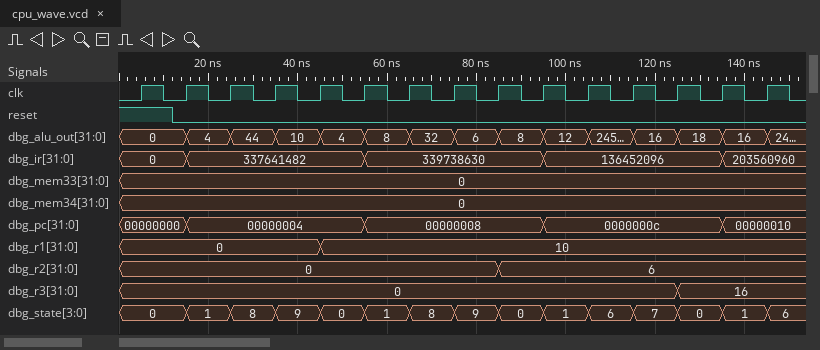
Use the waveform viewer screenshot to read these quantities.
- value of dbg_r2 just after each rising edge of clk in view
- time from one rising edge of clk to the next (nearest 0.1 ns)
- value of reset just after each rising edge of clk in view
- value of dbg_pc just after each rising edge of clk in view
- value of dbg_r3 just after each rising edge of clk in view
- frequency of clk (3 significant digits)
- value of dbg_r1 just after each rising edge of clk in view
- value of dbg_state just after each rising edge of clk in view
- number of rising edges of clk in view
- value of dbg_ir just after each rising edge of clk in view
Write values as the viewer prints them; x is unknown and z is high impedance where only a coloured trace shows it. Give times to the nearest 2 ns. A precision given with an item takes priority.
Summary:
0, 0, 0, 0, 0, 0, 0, 0, 6, 6, 6, 6, 6, 6, 6
10 ns
1 0 0 0 0 0 0 0 0 0 0 0 0 0 0
00000000, 00000004, 00000004, 00000004, 00000004, 00000008, 00000008, 00000008, 00000008, 0000000c, 0000000c, 0000000c, 0000000c, 00000010, 00000010
0, 0, 0, 0, 0, 0, 0, 0, 0, 0, 0, 0, 16, 16, 16
100 MHz
0, 0, 0, 0, 10, 10, 10, 10, 10, 10, 10, 10, 10, 10, 10
0, 1, 8, 9, 0, 1, 8, 9, 0, 1, 6, 7, 0, 1, 6
15
0, 337641482, 337641482, 337641482, 337641482, 339738630, 339738630, 339738630, 339738630, 136452096, 136452096, 136452096, 136452096, 203560960, 203560960
